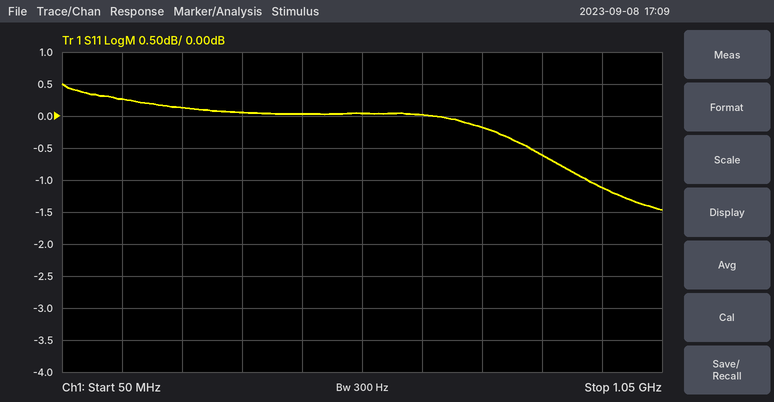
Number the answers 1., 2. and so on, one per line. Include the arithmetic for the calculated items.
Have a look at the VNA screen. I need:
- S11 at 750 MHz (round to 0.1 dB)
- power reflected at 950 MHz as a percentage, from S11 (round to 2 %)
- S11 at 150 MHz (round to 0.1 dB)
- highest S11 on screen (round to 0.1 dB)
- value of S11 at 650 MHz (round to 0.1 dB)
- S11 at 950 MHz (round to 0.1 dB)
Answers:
1. -0.2 dB
2. 10^(-1.1/10) ≈ 78 %
3. 0.3 dB
4. 0.5 dB
5. 0.0 dB
6. -1.1 dB
